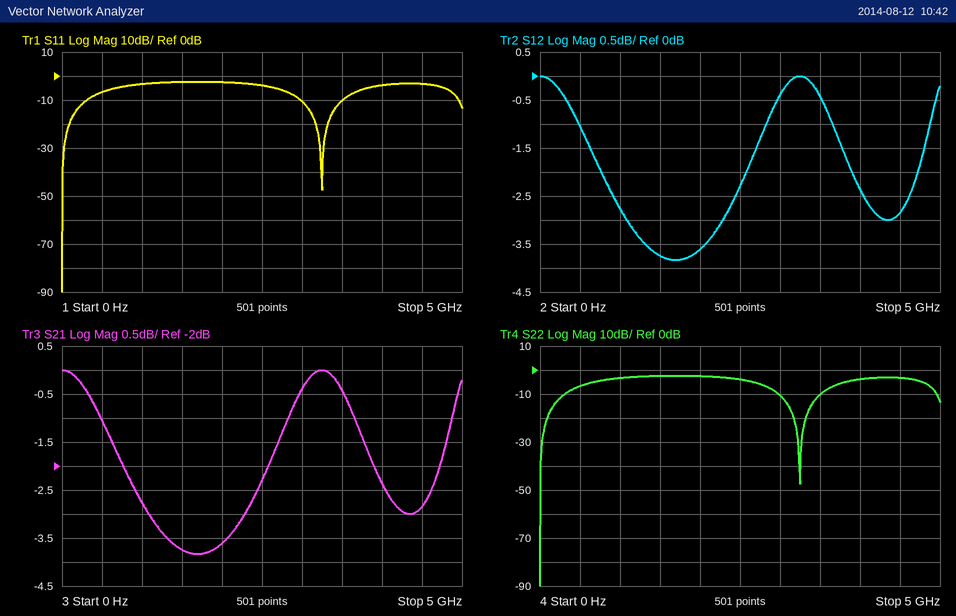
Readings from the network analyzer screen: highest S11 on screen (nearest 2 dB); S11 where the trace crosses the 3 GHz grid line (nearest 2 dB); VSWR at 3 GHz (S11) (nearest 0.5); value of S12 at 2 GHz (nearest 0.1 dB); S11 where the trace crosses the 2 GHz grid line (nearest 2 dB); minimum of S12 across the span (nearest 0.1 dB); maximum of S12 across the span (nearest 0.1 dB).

-2 dB
-10 dB
2.0
-3.6 dB
-2 dB
-3.8 dB
0.0 dB
